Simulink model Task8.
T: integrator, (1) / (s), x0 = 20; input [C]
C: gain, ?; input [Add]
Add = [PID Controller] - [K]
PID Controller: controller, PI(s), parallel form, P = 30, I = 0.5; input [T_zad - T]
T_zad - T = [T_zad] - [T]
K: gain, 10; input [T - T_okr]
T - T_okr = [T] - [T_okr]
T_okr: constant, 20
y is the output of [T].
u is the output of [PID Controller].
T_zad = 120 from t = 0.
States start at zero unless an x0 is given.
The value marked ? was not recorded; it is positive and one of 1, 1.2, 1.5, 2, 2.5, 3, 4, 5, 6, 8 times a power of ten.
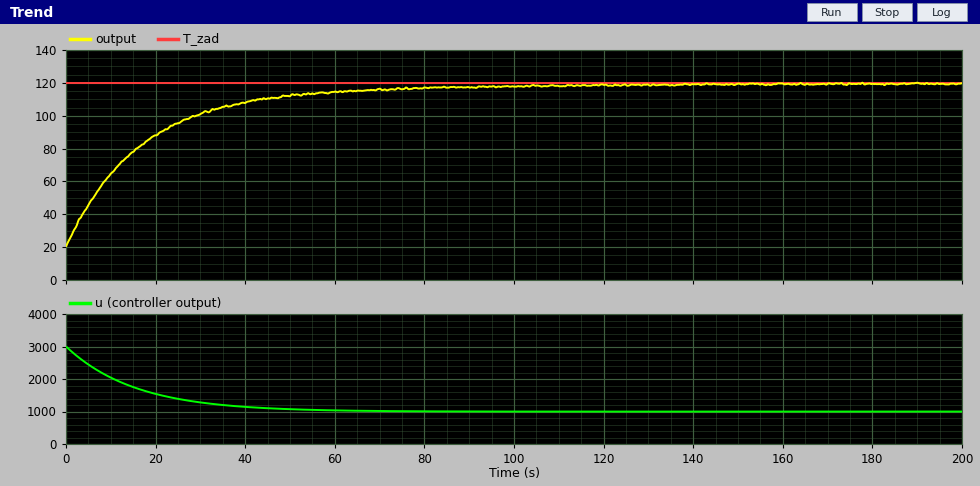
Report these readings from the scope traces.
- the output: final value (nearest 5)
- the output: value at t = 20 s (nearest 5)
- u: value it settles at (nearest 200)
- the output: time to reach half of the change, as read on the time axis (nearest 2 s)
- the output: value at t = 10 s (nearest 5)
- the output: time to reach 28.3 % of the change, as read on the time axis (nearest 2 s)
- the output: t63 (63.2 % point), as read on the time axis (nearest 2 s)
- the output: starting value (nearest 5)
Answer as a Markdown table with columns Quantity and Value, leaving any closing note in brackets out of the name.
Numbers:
| Quantity | Value |
|---|---|
| the output: final value | 120 |
| the output: value at t = 20 s | 90 |
| u: value it settles at | 1000 |
| the output: time to reach half of the change, as read on the time axis | 12 s |
| the output: value at t = 10 s | 65 |
| the output: time to reach 28.3 % of the change, as read on the time axis | 6 s |
| the output: t63 (63.2 % point), as read on the time axis | 18 s |
| the output: starting value | 20 |
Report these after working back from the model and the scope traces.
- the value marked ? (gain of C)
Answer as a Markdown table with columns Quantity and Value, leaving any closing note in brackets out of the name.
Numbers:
| Quantity | Value |
|---|---|
| the value marked ? | 0.002 |
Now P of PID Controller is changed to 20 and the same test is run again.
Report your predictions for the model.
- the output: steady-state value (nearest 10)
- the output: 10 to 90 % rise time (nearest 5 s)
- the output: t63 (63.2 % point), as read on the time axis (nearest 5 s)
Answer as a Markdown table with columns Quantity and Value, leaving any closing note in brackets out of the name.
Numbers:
| Quantity | Value |
|---|---|
| the output: steady-state value | 120 |
| the output: 10 to 90 % rise time | 45 s |
| the output: t63 (63.2 % point), as read on the time axis | 25 s |
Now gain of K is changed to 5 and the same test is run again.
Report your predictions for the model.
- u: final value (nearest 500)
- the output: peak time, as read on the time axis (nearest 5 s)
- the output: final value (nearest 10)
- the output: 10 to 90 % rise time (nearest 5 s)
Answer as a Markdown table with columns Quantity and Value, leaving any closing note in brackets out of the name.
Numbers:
| Quantity | Value |
|---|---|
| u: final value | 500 |
| the output: peak time, as read on the time axis | 75 s |
| the output: final value | 120 |
| the output: 10 to 90 % rise time | 30 s |
